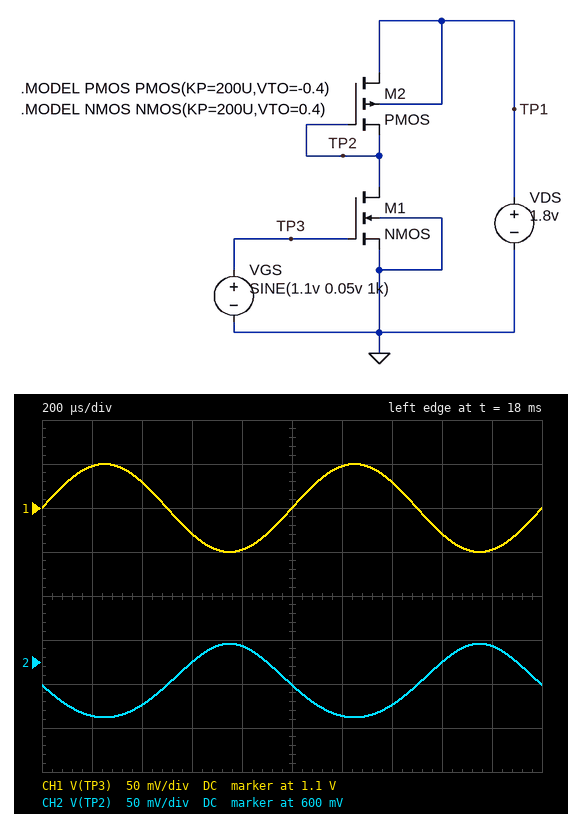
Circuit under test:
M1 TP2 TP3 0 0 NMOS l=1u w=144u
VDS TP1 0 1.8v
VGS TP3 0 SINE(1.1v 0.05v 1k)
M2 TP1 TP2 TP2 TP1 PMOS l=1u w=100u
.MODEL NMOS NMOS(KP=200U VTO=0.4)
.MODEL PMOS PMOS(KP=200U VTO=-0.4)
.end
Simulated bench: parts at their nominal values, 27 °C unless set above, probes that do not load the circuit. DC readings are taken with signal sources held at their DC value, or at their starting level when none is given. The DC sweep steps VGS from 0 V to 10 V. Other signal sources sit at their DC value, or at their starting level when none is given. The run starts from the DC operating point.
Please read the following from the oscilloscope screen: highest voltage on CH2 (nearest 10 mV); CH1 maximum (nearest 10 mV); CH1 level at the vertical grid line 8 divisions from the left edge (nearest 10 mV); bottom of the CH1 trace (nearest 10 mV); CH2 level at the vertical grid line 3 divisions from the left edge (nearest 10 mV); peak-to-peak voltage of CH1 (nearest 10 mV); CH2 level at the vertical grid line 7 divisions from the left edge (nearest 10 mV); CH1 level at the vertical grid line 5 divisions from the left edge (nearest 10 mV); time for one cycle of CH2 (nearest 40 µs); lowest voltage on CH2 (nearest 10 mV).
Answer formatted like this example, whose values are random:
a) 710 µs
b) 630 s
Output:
a) 620 mV
b) 1.15 V
c) 1.07 V
d) 1.05 V
e) 600 mV
f) 100 mV
g) 550 mV
h) 1.10 V
i) 1.00 ms
j) 540 mV
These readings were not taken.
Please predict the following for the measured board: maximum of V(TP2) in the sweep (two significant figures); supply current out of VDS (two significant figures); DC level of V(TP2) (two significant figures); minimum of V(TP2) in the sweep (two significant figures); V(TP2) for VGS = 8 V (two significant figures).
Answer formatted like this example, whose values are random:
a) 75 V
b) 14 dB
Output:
a) 1.4 V
b) 6.8 mA
c) 570 mV
d) 65 mV
e) 80 mV
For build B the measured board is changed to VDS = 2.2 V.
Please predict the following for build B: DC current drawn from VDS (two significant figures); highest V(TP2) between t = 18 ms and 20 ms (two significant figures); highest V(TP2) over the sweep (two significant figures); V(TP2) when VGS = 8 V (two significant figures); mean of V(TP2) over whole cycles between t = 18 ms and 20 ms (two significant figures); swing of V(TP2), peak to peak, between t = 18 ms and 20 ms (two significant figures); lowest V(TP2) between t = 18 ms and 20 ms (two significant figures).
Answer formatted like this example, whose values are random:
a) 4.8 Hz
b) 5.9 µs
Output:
a) 7.1 mA
b) 1.0 V
c) 1.8 V
d) 130 mV
e) 960 mV
f) 120 mV
g) 900 mV
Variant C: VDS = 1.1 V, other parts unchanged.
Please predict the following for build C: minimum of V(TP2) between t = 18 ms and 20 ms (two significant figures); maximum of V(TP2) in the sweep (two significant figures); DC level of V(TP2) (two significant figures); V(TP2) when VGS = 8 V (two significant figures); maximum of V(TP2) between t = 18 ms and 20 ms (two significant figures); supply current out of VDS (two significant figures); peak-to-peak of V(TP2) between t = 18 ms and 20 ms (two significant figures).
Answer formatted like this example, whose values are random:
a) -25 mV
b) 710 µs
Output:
a) 150 mV
b) 700 mV
c) 160 mV
d) 21 mV
e) 170 mV
f) 2.9 mA
g) 18 mV
